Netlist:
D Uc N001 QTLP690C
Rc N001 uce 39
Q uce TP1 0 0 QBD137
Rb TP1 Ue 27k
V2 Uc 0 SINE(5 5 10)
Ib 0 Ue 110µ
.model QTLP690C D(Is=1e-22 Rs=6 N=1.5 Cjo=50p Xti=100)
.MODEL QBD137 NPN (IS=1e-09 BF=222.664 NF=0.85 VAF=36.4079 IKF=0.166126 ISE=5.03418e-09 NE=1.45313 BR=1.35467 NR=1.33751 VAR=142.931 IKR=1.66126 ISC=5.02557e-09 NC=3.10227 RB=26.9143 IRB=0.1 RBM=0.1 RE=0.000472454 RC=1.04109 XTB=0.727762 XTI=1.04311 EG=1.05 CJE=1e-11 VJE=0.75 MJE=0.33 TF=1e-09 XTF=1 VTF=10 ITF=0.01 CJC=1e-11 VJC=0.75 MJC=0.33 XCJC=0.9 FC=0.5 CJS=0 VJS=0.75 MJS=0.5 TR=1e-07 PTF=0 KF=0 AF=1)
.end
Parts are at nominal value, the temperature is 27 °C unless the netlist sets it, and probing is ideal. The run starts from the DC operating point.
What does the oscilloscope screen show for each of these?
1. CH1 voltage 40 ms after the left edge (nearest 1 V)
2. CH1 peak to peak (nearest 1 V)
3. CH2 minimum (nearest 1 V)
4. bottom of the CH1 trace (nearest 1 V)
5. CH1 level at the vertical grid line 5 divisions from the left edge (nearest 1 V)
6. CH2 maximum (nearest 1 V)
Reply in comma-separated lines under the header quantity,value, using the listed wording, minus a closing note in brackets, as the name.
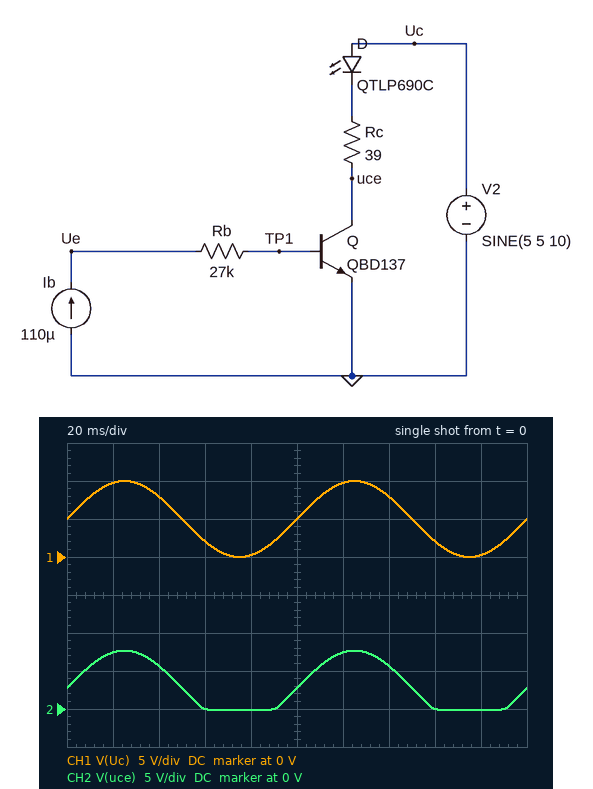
quantity,value
CH1 voltage 40 ms after the left edge,8 V
CH1 peak to peak,10 V
CH2 minimum,0 V
bottom of the CH1 trace,0 V
CH1 level at the vertical grid line 5 divisions from the left edge,5 V
CH2 maximum,8 V
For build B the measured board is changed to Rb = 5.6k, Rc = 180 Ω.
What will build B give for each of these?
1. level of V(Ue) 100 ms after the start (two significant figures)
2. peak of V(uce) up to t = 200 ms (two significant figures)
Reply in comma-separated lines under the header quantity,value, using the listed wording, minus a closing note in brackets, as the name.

quantity,value
level of V(Ue) 100 ms after the start,970 mV
peak of V(uce) up to t = 200 ms,6.1 V
